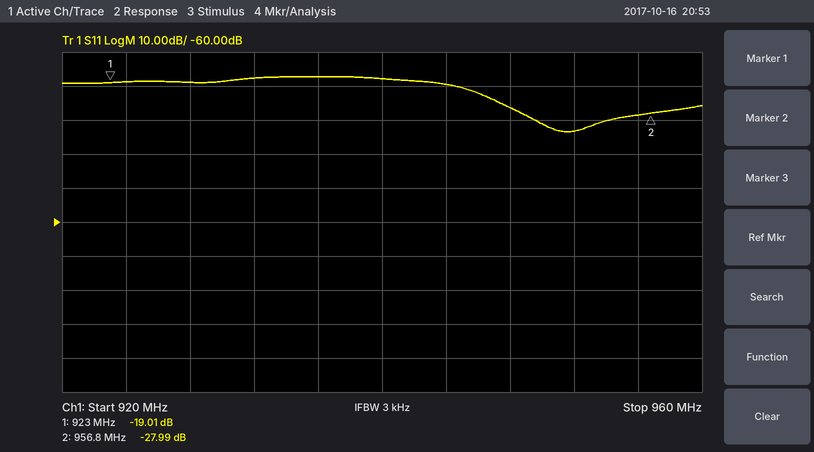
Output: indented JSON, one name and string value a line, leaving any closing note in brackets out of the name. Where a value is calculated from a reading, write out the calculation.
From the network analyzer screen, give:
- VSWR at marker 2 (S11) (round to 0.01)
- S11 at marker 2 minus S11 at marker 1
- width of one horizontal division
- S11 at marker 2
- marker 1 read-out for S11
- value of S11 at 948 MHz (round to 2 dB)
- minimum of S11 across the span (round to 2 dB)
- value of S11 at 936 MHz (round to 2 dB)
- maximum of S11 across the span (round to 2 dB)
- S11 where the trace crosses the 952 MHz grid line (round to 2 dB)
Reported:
{
  "VSWR at marker 2 (S11)": "(1 + 0.0399)/(1 − 0.0399) ≈ 1.08",
  "S11 at marker 2 minus S11 at marker 1": "-27.99 − (-19.01) = -8.98 dB",
  "width of one horizontal division": "4 MHz",
  "S11 at marker 2": "-27.99 dB",
  "marker 1 read-out for S11": "-19.01 dB",
  "value of S11 at 948 MHz": "-26 dB",
  "minimum of S11 across the span": "-34 dB",
  "value of S11 at 936 MHz": "-18 dB",
  "maximum of S11 across the span": "-18 dB",
  "S11 where the trace crosses the 952 MHz grid line": "-34 dB"
}
